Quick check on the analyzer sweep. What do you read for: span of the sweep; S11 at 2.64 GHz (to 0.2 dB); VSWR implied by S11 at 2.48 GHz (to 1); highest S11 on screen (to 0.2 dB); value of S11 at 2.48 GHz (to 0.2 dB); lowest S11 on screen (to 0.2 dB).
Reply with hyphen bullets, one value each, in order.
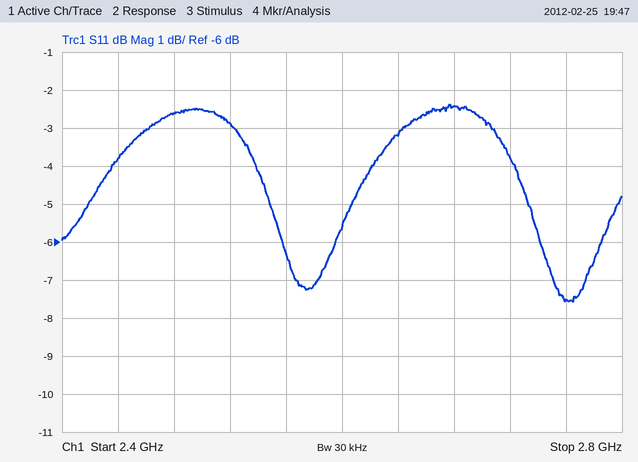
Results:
- 400 MHz
- -3.2 dB
- 7
- -2.4 dB
- -2.6 dB
- -7.6 dB
